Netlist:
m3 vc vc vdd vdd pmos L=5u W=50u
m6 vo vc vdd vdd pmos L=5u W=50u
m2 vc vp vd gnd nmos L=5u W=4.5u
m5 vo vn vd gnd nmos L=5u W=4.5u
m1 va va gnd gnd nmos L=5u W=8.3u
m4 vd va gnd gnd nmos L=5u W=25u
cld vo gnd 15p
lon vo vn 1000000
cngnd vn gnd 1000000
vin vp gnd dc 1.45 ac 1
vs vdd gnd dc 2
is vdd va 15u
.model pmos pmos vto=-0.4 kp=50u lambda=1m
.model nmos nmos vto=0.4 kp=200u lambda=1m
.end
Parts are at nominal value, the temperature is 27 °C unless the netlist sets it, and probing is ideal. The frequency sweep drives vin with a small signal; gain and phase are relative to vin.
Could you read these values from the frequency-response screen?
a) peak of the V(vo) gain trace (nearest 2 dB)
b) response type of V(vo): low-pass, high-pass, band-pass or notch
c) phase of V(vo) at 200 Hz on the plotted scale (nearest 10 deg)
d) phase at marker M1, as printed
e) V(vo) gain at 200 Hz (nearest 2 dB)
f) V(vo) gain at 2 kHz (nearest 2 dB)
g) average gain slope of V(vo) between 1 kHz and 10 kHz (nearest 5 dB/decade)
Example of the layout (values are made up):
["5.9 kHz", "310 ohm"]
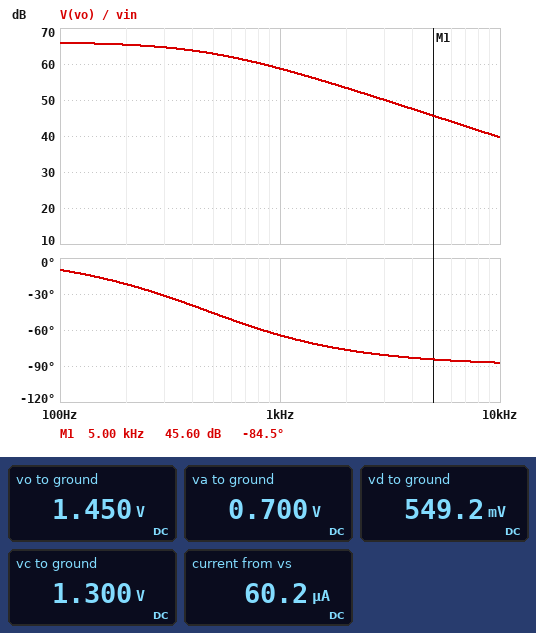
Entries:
["66 dB", "low-pass", "-20 deg", "-84.5 deg", "66 dB", "54 dB", "-20 dB/decade"]
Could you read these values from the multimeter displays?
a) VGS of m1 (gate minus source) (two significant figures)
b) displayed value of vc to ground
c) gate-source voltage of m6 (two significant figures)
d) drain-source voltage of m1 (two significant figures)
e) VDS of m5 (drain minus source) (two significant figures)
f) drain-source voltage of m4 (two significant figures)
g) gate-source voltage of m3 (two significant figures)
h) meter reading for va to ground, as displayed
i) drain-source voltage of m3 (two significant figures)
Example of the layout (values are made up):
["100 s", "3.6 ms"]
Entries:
["700 mV", "1.300 V", "-700 mV", "700 mV", "900 mV", "550 mV", "-700 mV", "0.700 V", "-700 mV"]
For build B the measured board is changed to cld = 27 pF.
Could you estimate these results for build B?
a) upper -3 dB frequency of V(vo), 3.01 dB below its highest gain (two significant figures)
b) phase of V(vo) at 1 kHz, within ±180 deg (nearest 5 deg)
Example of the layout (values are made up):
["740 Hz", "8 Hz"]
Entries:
["270 Hz", "-75 deg"]
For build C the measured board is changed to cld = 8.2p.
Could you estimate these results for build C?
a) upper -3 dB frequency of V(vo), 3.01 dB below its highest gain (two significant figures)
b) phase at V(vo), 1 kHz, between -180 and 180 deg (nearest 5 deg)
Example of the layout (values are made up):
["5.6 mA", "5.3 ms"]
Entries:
["880 Hz", "-50 deg"]
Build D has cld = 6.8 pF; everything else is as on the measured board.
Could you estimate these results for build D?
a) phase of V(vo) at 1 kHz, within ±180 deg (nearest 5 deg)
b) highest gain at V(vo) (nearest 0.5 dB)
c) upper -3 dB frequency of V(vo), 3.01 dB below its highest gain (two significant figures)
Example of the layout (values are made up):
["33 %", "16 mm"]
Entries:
["-45 deg", "66.0 dB", "1.1 kHz"]
